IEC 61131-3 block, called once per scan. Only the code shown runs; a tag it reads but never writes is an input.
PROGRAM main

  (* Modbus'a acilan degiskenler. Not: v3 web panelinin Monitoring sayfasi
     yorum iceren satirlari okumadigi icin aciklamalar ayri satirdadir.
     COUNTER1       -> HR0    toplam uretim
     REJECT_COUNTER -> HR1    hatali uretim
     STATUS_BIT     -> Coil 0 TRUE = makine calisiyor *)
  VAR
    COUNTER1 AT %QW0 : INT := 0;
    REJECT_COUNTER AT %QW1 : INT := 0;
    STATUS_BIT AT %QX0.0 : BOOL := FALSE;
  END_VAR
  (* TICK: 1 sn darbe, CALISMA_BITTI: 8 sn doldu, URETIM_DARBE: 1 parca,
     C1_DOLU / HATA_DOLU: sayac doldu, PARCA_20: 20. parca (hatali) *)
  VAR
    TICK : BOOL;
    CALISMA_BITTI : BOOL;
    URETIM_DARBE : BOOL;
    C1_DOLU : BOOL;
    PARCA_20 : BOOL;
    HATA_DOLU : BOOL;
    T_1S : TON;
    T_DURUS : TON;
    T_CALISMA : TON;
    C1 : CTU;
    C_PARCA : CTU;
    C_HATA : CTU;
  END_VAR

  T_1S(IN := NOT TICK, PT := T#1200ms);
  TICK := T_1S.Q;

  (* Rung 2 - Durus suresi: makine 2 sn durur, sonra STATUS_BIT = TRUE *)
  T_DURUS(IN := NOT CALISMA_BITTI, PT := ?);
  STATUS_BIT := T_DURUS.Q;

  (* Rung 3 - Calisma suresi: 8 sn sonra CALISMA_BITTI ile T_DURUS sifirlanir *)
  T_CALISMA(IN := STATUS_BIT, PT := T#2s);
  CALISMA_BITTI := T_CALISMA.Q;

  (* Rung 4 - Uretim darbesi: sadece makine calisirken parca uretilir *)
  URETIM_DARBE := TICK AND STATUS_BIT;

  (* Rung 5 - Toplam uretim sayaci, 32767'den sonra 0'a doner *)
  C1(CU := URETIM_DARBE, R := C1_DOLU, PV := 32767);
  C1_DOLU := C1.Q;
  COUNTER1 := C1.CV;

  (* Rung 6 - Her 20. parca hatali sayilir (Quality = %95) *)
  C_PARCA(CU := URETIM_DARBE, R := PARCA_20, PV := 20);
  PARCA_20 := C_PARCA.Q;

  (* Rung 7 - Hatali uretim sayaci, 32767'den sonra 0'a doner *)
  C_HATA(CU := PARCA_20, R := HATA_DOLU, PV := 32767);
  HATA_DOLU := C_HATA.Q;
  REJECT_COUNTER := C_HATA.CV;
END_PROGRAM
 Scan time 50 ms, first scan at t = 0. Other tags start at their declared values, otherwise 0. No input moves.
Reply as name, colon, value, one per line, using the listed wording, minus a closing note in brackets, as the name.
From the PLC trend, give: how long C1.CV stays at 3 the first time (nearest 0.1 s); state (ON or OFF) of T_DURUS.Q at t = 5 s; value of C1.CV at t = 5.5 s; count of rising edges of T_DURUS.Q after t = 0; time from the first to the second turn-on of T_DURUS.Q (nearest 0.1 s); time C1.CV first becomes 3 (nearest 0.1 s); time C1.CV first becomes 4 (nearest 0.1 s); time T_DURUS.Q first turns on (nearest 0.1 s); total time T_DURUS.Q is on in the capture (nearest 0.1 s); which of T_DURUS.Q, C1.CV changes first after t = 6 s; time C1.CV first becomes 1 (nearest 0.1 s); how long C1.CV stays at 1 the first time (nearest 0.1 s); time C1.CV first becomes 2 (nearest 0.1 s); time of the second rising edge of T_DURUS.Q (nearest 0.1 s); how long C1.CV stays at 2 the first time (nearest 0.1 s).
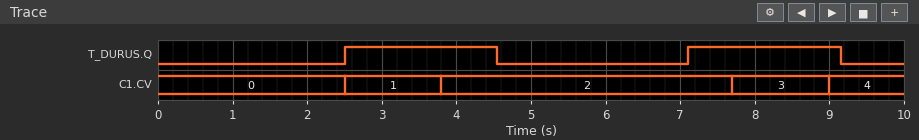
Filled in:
how long C1.CV stays at 3 the first time: 1.3 s
state (ON or OFF) of T_DURUS.Q at t = 5 s: OFF
value of C1.CV at t = 5.5 s: 2
count of rising edges of T_DURUS.Q after t = 0: 2
time from the first to the second turn-on of T_DURUS.Q: 4.6 s
time C1.CV first becomes 3: 7.7 s
time C1.CV first becomes 4: 9.0 s
time T_DURUS.Q first turns on: 2.5 s
total time T_DURUS.Q is on in the capture: 4.1 s
which of T_DURUS.Q, C1.CV changes first after t = 6 s: T_DURUS.Q
time C1.CV first becomes 1: 2.5 s
how long C1.CV stays at 1 the first time: 1.3 s
time C1.CV first becomes 2: 3.8 s
time of the second rising edge of T_DURUS.Q: 7.1 s
how long C1.CV stays at 2 the first time: 3.9 s
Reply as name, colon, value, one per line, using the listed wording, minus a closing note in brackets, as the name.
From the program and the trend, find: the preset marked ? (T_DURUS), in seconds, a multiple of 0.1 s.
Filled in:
the preset marked ? (T_DURUS), in seconds, a multiple of 0.1 s: 2.5 s
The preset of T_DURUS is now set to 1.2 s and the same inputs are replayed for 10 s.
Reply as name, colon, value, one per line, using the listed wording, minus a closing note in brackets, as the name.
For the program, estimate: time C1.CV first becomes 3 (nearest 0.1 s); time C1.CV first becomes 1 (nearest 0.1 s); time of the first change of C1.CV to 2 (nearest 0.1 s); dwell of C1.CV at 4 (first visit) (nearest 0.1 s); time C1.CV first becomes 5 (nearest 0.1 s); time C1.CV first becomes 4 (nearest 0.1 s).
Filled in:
time C1.CV first becomes 3: 5.1 s
time C1.CV first becomes 1: 1.2 s
time of the first change of C1.CV to 2: 2.5 s
dwell of C1.CV at 4 (first visit): 2.6 s
time C1.CV first becomes 5: 9.0 s
time C1.CV first becomes 4: 6.4 s
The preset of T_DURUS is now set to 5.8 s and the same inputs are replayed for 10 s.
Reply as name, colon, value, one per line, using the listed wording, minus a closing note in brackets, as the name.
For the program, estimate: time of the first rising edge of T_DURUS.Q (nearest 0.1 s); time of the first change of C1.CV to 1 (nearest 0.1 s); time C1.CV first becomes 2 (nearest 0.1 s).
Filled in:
time of the first rising edge of T_DURUS.Q: 5.8 s
time of the first change of C1.CV to 1: 6.4 s
time C1.CV first becomes 2: 7.7 s
